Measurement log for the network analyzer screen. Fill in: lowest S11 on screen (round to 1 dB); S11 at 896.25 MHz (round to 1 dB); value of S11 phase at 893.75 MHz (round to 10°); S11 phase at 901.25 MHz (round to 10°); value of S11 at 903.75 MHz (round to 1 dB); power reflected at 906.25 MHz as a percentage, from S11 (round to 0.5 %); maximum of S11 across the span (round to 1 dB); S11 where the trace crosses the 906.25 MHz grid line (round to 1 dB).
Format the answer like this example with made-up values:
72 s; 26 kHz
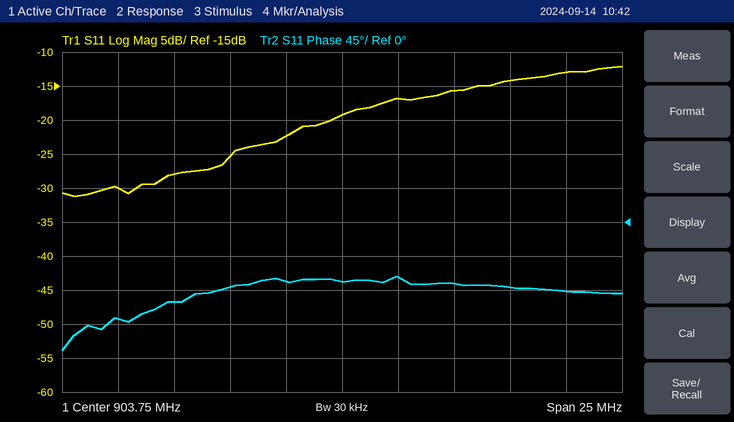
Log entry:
-31 dB; -28 dB; -130°; -80°; -19 dB; 2.0 %; -12 dB; -17 dB
